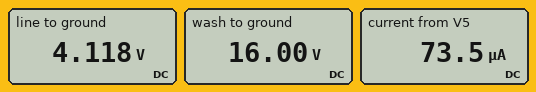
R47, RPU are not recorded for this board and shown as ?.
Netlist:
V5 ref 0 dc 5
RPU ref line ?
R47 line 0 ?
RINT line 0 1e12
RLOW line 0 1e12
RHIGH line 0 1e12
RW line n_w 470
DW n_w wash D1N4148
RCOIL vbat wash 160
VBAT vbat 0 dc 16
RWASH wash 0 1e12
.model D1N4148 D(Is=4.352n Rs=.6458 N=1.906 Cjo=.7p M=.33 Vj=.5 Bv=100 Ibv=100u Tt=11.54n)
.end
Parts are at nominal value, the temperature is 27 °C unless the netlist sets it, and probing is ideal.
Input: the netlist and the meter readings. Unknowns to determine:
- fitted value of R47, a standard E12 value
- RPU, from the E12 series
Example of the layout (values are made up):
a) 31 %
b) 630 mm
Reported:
a) 56 kΩ
b) 12 kΩ
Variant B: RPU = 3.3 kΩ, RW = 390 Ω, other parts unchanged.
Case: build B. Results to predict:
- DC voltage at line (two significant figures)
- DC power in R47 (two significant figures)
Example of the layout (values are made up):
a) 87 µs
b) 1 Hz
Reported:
a) 4.7 V
b) 400 µW
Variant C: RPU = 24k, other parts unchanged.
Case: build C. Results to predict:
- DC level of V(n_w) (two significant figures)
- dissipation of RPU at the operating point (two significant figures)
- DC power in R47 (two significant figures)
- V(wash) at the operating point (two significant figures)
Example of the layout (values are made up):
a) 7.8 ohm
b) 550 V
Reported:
a) 3.5 V
b) 94 µW
c) 220 µW
d) 16 V
